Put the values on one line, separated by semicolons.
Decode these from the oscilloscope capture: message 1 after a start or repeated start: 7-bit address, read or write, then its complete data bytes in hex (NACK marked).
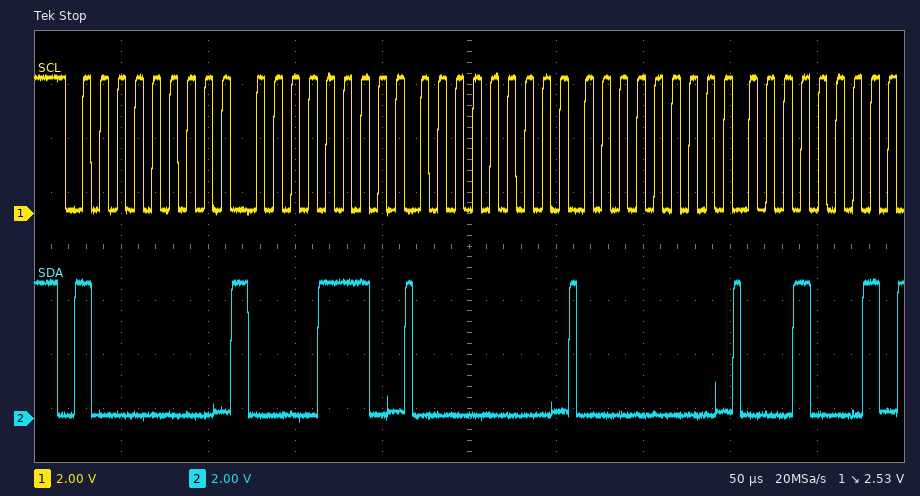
0x40 write: 0E 00 00 11
